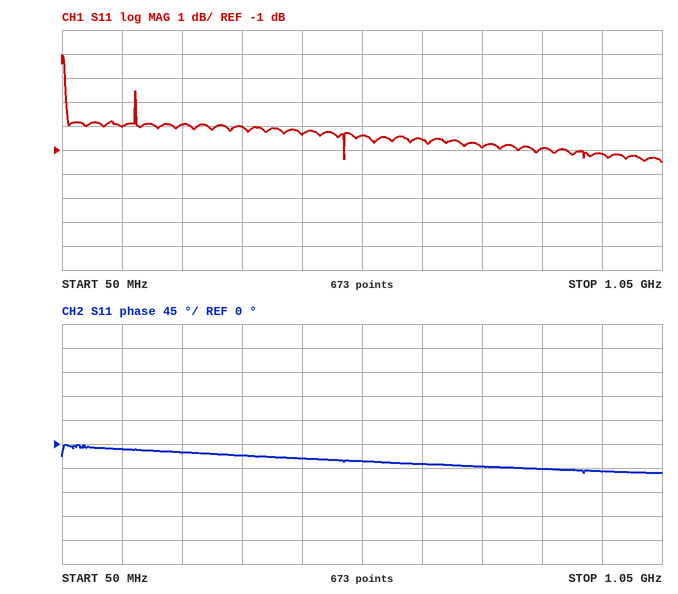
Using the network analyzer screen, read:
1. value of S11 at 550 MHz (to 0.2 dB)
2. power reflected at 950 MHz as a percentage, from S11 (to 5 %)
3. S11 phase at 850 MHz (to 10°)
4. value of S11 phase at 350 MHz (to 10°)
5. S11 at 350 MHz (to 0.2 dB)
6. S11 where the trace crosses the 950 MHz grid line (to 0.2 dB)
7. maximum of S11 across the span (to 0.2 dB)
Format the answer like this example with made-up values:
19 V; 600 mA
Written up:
-0.4 dB; 75 %; -50°; -20°; 0.0 dB; -1.2 dB; 3.0 dB
